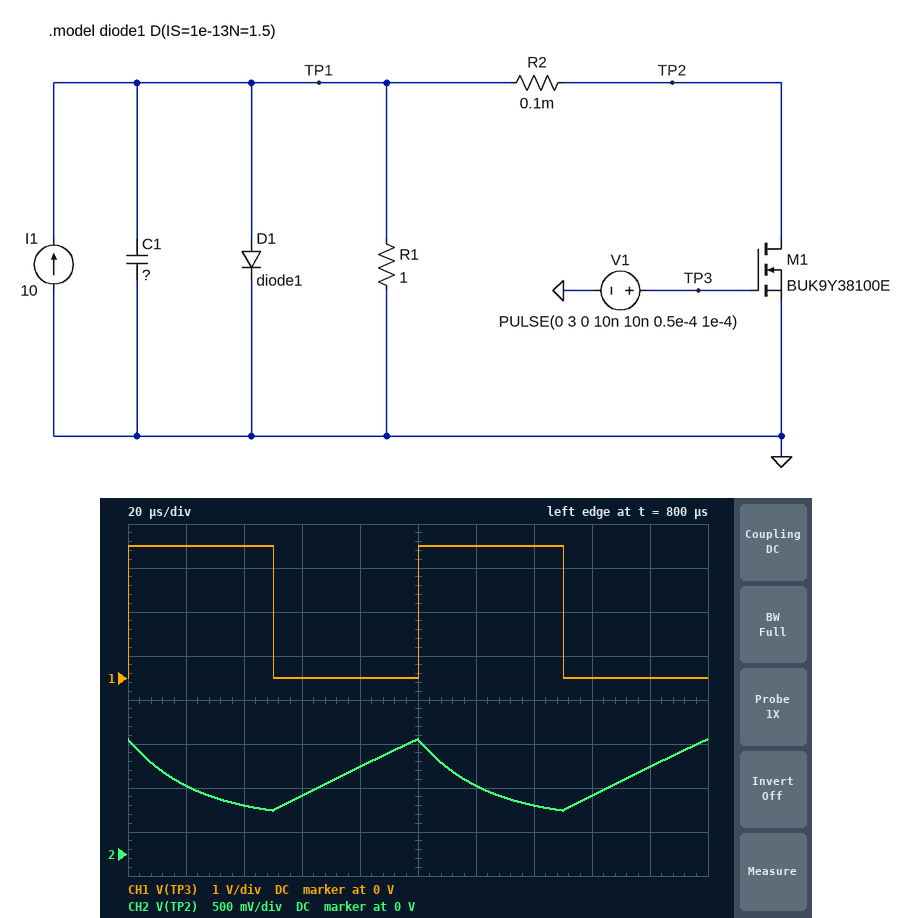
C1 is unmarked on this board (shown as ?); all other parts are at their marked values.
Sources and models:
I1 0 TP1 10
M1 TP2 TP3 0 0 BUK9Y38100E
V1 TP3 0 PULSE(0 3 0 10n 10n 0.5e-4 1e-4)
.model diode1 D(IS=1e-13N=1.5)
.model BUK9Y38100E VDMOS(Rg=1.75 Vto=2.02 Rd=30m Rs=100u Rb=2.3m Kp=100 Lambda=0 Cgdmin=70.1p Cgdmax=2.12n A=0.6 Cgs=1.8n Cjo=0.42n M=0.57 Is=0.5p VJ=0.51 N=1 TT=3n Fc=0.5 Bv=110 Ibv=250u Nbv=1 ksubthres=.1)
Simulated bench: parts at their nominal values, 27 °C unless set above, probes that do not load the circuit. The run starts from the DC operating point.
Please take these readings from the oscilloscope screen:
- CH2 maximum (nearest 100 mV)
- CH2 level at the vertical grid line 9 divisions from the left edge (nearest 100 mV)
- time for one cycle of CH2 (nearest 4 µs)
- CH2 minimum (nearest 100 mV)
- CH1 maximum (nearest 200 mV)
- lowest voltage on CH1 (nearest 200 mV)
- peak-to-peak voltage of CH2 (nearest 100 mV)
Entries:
1.3 V
1.0 V
100 µs
500 mV
3.0 V
0 V
800 mV
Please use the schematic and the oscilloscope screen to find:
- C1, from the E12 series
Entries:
560 µF
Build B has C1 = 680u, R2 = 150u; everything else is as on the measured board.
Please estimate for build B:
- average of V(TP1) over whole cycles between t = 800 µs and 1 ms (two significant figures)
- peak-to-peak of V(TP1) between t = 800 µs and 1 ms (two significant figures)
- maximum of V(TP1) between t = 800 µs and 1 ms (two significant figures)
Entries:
820 mV
670 mV
1.2 V
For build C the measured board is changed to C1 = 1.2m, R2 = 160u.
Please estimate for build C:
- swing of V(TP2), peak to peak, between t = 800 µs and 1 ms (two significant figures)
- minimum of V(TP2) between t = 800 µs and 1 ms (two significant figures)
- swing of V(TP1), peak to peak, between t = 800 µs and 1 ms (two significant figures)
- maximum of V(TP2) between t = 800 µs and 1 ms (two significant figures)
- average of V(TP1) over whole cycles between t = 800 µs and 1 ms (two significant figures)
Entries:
390 mV
610 mV
380 mV
990 mV
790 mV
